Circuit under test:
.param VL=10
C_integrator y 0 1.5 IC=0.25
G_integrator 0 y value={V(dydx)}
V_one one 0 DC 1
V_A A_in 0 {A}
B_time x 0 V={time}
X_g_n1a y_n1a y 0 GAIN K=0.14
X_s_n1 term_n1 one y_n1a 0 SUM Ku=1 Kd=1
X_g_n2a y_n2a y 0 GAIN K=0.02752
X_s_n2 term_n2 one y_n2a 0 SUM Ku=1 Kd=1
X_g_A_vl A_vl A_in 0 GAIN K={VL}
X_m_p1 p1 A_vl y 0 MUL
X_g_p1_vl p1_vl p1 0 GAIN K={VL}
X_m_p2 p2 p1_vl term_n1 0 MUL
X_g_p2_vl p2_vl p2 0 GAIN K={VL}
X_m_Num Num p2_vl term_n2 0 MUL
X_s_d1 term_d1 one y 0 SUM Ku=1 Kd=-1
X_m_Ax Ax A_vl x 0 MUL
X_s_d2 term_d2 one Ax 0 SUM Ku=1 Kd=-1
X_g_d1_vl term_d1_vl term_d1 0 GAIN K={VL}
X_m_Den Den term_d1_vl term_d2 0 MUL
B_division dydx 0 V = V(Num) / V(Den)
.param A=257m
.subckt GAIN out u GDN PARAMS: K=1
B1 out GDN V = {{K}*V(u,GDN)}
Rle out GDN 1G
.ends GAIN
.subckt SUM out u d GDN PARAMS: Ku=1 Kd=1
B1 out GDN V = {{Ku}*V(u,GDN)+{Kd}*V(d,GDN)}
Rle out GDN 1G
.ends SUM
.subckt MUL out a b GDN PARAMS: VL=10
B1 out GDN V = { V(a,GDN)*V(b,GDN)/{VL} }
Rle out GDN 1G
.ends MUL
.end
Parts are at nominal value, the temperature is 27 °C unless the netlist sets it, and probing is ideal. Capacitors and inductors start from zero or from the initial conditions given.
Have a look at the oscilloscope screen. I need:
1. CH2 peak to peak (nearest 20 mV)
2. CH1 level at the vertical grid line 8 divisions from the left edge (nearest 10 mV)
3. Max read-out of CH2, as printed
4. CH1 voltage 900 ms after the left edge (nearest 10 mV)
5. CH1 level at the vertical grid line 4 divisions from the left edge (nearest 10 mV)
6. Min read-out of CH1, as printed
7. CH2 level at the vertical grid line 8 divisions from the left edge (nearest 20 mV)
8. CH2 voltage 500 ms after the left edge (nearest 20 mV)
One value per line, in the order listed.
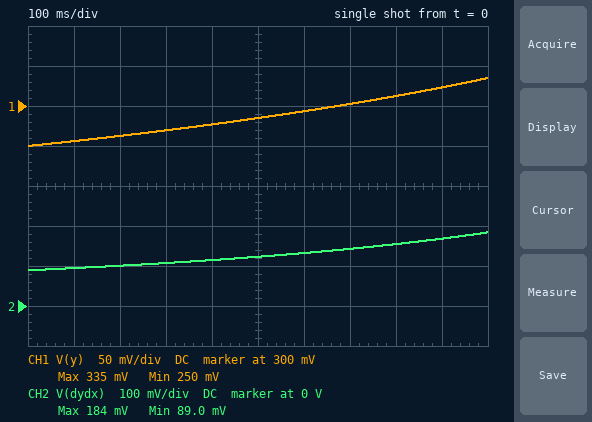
100 mV
310 mV
184 mV
320 mV
280 mV
250 mV
160 mV
120 mV
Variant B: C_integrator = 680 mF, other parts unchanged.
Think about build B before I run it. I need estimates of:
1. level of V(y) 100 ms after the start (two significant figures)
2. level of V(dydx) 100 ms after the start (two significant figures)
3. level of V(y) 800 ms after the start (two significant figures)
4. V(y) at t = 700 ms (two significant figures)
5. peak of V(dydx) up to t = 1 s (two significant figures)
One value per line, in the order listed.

260 mV
99 mV
430 mV
390 mV
410 mV
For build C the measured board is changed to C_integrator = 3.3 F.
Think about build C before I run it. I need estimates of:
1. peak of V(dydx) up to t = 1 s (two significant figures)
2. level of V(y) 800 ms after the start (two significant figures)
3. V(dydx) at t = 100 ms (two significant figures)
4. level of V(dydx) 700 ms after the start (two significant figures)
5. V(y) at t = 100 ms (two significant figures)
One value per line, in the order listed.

140 mV
280 mV
93 mV
120 mV
250 mV
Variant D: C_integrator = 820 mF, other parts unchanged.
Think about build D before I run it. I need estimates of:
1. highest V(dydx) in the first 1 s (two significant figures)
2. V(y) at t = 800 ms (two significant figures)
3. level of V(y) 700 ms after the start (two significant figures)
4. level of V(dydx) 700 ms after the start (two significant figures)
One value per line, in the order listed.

300 mV
380 mV
360 mV
190 mV
